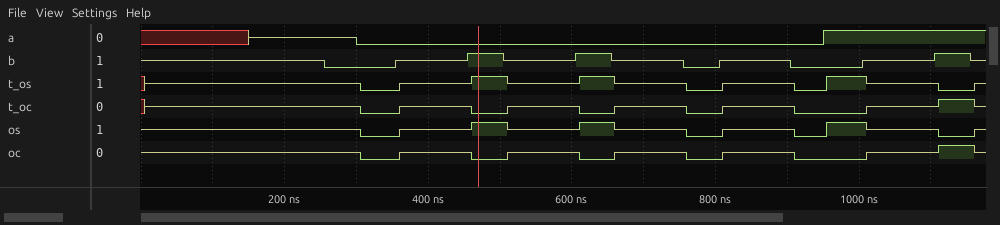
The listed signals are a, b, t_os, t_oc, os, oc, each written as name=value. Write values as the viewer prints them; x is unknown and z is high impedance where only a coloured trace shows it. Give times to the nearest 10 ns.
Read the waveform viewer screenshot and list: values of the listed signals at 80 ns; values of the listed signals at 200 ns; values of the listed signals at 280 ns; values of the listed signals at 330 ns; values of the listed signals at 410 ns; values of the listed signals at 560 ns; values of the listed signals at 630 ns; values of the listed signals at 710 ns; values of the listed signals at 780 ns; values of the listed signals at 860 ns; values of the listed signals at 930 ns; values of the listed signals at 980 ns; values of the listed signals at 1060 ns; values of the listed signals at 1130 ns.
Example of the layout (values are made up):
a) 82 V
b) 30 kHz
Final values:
a) a=x, b=z, t_os=z, t_oc=z, os=z, oc=z
b) a=z, b=z, t_os=z, t_oc=z, os=z, oc=z
c) a=z, b=0, t_os=z, t_oc=z, os=z, oc=z
d) a=0, b=0, t_os=0, t_oc=0, os=0, oc=0
e) a=0, b=z, t_os=z, t_oc=z, os=z, oc=z
f) a=0, b=z, t_os=z, t_oc=z, os=z, oc=z
g) a=0, b=1, t_os=1, t_oc=0, os=1, oc=0
h) a=0, b=z, t_os=z, t_oc=z, os=z, oc=z
i) a=0, b=0, t_os=0, t_oc=0, os=0, oc=0
j) a=0, b=z, t_os=z, t_oc=z, os=z, oc=z
k) a=0, b=0, t_os=0, t_oc=0, os=0, oc=0
l) a=1, b=0, t_os=1, t_oc=0, os=1, oc=0
m) a=1, b=z, t_os=z, t_oc=z, os=z, oc=z
n) a=1, b=1, t_os=0, t_oc=1, os=0, oc=1
